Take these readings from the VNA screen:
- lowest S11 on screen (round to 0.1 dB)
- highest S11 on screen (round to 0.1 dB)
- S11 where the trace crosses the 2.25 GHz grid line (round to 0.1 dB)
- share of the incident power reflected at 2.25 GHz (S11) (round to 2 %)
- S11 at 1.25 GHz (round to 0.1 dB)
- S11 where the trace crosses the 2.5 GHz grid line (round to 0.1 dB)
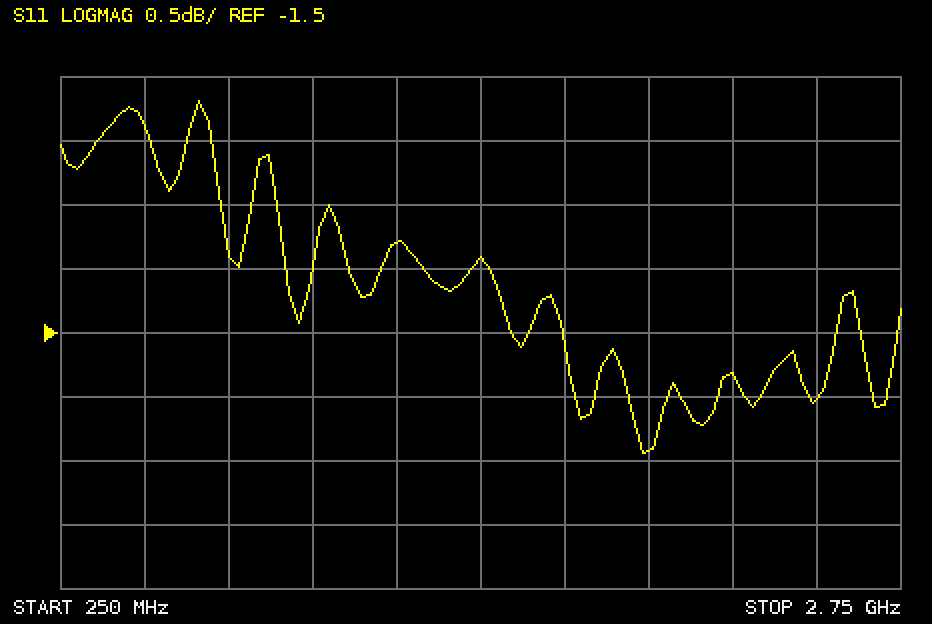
-2.4 dB
0.3 dB
-1.8 dB
66 %
-0.8 dB
-2.0 dB
